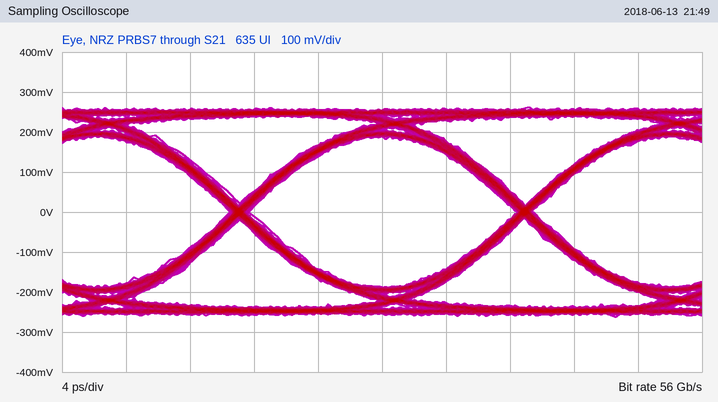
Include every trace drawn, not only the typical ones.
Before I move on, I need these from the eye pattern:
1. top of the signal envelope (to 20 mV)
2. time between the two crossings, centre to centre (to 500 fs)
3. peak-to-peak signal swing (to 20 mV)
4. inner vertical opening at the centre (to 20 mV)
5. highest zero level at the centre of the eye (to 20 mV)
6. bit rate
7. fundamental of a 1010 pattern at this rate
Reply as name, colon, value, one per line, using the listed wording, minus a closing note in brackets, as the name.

top of the signal envelope: 260 mV
time between the two crossings, centre to centre: 18.0 ps
peak-to-peak signal swing: 520 mV
inner vertical opening at the centre: 380 mV
highest zero level at the centre of the eye: -180 mV
bit rate: 56 Gb/s
fundamental of a 1010 pattern at this rate: 28 GHz
